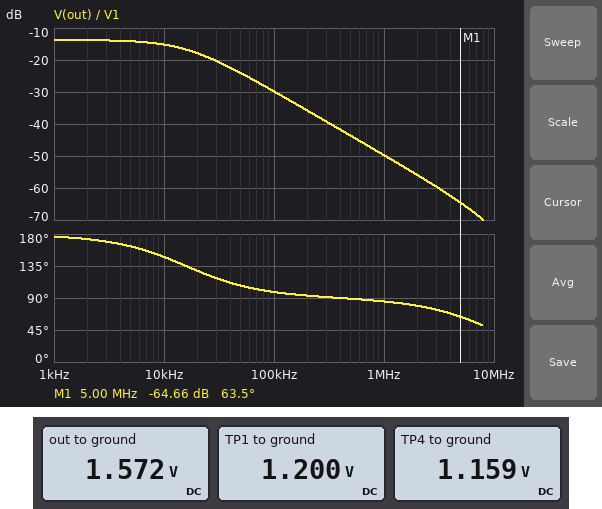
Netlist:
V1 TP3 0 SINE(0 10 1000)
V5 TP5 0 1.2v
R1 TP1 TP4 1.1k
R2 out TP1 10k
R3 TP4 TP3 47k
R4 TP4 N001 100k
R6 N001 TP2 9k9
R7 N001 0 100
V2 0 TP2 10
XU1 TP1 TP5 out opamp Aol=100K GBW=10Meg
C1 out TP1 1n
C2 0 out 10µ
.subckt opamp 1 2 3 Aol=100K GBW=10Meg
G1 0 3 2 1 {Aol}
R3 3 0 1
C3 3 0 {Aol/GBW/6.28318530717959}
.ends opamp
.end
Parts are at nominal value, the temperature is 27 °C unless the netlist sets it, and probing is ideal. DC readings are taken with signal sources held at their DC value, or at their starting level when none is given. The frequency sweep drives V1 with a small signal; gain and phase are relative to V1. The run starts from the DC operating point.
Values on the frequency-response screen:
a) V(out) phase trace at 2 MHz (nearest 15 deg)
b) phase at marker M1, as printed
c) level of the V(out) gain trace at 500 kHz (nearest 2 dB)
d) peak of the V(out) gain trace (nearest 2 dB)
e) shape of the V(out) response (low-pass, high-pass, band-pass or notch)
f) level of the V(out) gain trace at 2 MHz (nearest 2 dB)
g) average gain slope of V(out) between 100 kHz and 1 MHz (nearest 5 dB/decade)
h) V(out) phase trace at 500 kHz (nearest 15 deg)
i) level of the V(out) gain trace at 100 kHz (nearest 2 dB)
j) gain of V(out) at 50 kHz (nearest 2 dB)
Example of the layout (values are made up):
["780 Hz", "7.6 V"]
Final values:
["75 deg", "63.5 deg", "-44 dB", "-14 dB", "low-pass", "-56 dB", "-20 dB/decade", "90 deg", "-30 dB", "-24 dB"]
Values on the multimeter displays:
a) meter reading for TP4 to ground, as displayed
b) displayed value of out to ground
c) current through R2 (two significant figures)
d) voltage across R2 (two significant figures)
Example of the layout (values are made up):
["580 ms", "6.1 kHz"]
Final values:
["1.159 V", "1.572 V", "37 µA", "370 mV"]
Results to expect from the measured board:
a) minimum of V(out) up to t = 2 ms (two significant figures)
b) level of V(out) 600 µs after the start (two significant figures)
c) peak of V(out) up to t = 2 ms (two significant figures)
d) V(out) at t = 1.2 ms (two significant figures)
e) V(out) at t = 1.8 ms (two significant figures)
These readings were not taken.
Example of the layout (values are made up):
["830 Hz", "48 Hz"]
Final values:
["-480 mV", "2.7 V", "3.6 V", "-340 mV", "3.6 V"]
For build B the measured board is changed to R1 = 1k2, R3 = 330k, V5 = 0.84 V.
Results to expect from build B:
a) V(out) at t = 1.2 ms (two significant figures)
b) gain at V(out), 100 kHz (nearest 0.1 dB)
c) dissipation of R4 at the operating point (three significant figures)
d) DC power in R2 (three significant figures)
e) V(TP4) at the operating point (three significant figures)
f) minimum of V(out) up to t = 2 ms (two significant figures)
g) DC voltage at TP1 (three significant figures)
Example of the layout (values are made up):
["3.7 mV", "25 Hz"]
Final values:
["680 mV", "-46.6 dB", "8.56 µW", "1.38 µW", "826 mV", "660 mV", "840 mV"]
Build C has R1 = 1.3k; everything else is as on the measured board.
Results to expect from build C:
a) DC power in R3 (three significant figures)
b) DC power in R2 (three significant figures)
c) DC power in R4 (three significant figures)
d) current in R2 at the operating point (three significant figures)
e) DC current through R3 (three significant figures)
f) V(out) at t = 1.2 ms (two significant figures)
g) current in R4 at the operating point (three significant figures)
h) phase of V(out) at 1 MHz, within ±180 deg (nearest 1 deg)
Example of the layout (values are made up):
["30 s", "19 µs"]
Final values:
["28.2 µW", "13.7 µW", "15.6 µW", "37.0 µA", "24.5 µA", "-330 mV", "12.5 µA", "85 deg"]
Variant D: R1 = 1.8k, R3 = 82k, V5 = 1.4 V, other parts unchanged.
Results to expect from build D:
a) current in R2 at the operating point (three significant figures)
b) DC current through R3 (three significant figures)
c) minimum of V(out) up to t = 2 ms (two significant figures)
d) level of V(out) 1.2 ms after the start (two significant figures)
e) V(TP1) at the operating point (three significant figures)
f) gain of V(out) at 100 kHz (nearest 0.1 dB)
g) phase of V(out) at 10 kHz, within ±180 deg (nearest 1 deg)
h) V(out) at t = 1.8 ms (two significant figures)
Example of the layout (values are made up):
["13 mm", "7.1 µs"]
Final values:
["30.8 µA", "16.4 µA", "540 mV", "620 mV", "1.40 V", "-34.7 dB", "148 deg", "2.8 V"]
